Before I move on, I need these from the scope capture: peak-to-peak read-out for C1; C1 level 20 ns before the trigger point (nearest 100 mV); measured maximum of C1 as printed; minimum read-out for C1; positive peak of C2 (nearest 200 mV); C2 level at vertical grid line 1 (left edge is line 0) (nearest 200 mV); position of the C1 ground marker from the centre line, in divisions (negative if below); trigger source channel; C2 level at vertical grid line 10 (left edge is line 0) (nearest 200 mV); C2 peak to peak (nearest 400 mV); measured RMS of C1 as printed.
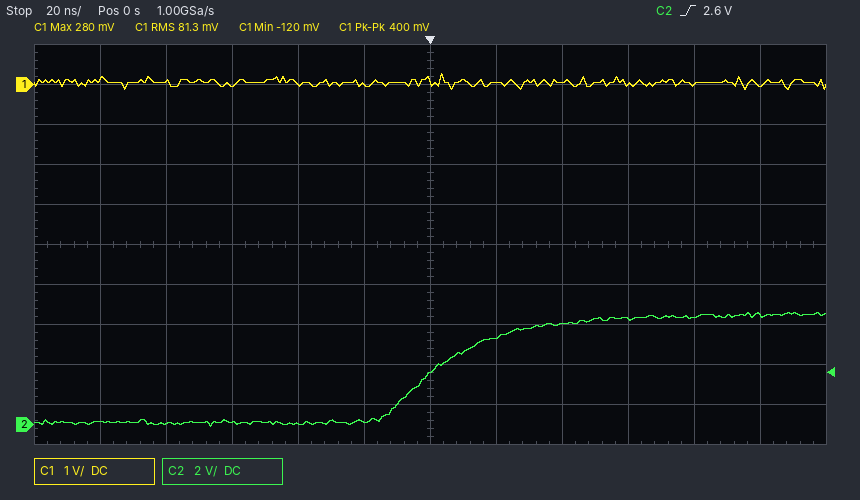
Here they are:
400 mV
0.0 V
280 mV
-120 mV
5.6 V
200 mV
+4.0 div
C2
5.4 V
5.6 V
81.3 mV
